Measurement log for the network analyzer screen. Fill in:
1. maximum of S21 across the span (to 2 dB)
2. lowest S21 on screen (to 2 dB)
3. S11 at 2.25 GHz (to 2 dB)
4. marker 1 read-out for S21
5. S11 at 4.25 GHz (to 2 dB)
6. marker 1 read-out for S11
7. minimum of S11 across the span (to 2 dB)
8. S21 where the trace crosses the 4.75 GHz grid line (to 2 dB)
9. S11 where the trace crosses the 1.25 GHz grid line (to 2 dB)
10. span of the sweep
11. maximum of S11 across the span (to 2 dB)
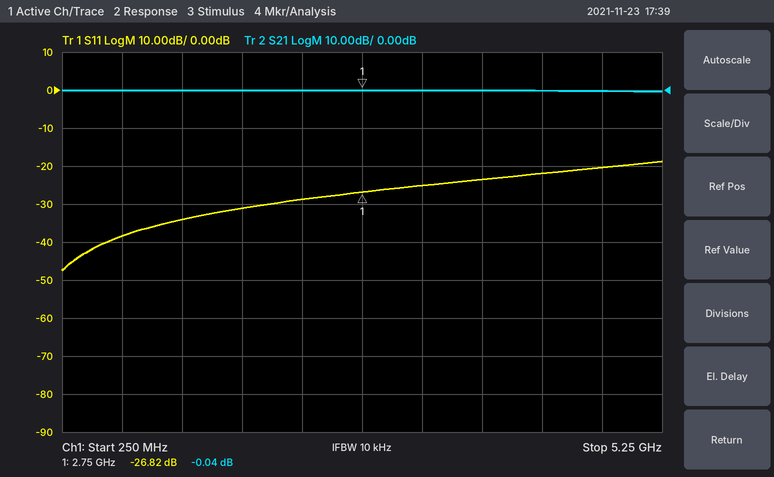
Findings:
0 dB
0 dB
-28 dB
-0.04 dB
-22 dB
-26.82 dB
-48 dB
0 dB
-34 dB
5 GHz
-18 dB
